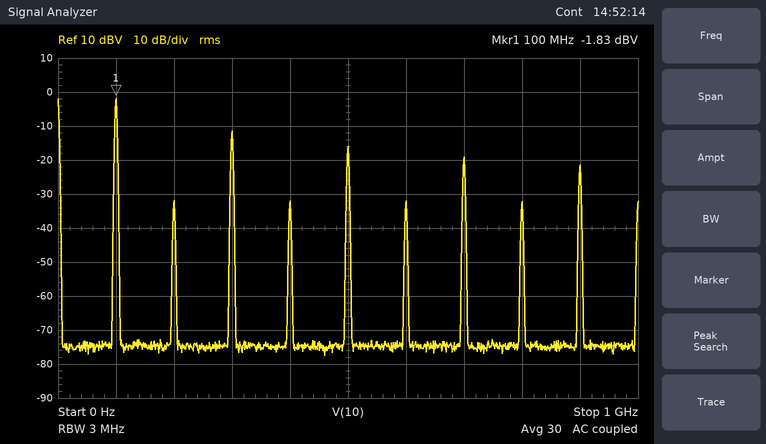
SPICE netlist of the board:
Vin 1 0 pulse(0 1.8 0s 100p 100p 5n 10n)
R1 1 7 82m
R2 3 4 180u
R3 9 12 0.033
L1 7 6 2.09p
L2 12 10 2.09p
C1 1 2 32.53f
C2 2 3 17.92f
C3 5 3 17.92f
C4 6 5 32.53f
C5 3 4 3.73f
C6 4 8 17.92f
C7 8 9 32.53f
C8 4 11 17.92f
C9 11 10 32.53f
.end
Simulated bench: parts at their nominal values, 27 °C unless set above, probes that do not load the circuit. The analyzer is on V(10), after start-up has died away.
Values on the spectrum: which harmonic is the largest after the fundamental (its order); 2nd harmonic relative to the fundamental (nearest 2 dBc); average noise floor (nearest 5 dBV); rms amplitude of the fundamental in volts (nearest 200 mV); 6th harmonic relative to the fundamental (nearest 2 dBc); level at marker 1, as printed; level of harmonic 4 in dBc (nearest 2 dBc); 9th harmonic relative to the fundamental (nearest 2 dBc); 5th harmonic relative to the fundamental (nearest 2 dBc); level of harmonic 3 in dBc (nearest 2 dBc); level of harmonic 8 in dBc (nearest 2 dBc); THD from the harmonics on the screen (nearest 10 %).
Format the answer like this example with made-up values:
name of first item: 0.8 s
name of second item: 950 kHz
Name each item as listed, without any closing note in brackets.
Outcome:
which harmonic is the largest after the fundamental: 3
2nd harmonic relative to the fundamental: -30 dBc
average noise floor: -75 dBV
rms amplitude of the fundamental in volts: 800 mV
6th harmonic relative to the fundamental: -30 dBc
level at marker 1, as printed: -1.83 dBV
level of harmonic 4 in dBc: -30 dBc
9th harmonic relative to the fundamental: -20 dBc
5th harmonic relative to the fundamental: -14 dBc
level of harmonic 3 in dBc: -10 dBc
level of harmonic 8 in dBc: -30 dBc
THD from the harmonics on the screen: 40 %
